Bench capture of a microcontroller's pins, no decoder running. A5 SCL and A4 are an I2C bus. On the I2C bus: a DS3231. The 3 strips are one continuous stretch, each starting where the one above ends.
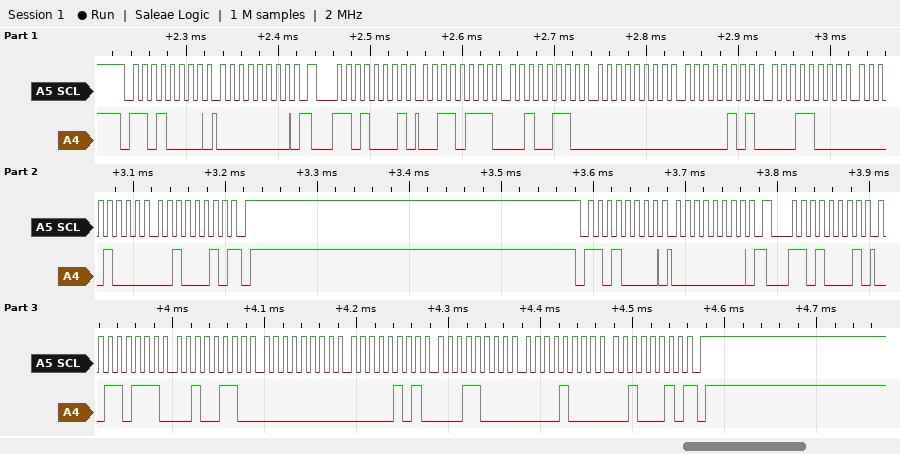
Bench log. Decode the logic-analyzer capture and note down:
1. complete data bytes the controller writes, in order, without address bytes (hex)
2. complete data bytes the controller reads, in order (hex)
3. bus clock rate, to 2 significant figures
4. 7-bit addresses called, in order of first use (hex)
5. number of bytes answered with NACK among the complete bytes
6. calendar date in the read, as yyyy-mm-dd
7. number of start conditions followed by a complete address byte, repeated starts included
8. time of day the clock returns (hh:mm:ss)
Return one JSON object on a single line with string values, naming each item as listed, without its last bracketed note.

{"complete data bytes the controller writes, in order, without address bytes": "00 00", "complete data bytes the controller reads, in order": "37 26 00 05 18 08 22 37 26 00 05 18 08 22", "bus clock rate, to 2 significant figures": "100 kHz", "7-bit addresses called, in order of first use": "0x68", "number of bytes answered with NACK among the complete bytes": "2", "calendar date in the read, as yyyy-mm-dd": "2022-08-18", "number of start conditions followed by a complete address byte, repeated starts included": "4", "time of day the clock returns": "00:26:37"}
